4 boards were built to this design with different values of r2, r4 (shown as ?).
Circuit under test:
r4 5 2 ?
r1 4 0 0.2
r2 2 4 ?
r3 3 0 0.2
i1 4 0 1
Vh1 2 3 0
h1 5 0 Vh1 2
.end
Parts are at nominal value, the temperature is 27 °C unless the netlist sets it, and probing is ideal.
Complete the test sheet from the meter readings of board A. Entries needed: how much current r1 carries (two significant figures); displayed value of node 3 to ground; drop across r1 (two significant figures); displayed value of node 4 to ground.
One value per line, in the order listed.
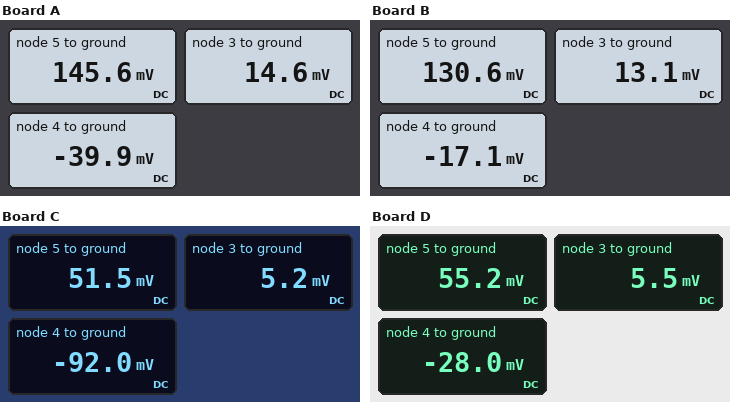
200 mA
14.6 mV
40 mV
-39.9 mV
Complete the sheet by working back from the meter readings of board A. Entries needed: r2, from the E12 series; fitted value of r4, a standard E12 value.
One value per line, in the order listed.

0.068 Ω
0.15 Ω
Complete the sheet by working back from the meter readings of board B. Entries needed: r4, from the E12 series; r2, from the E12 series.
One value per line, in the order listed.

0.12 Ω
0.033 Ω
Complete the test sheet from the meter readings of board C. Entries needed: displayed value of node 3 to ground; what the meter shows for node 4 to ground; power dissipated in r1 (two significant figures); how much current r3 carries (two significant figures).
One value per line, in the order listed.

5.2 mV
-92.0 mV
42 mW
26 mA
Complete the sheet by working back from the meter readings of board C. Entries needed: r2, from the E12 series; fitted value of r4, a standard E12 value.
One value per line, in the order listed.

0.18 Ω
0.082 Ω
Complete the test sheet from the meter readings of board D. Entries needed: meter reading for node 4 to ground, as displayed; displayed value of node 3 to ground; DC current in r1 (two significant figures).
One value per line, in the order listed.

-28.0 mV
5.5 mV
140 mA
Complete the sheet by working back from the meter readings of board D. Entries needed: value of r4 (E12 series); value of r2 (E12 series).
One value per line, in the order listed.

0.056 Ω
0.039 Ω
